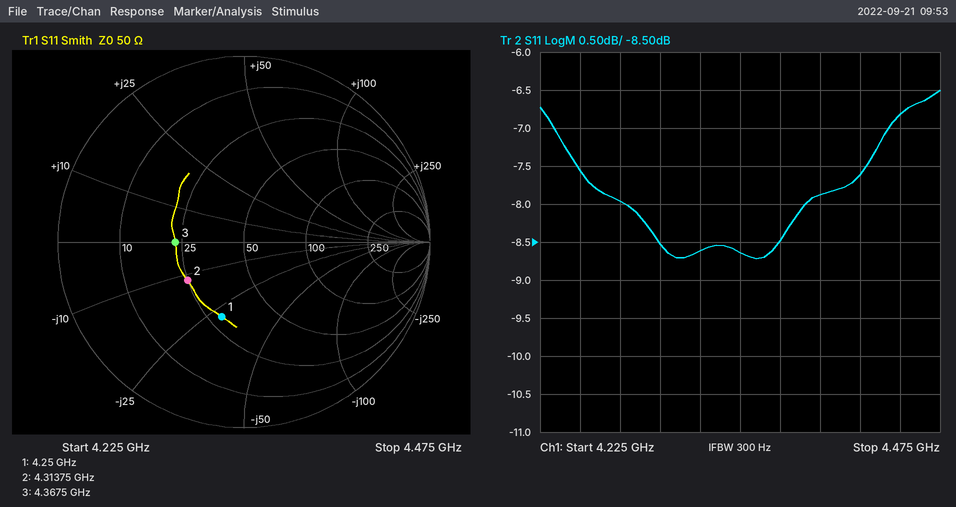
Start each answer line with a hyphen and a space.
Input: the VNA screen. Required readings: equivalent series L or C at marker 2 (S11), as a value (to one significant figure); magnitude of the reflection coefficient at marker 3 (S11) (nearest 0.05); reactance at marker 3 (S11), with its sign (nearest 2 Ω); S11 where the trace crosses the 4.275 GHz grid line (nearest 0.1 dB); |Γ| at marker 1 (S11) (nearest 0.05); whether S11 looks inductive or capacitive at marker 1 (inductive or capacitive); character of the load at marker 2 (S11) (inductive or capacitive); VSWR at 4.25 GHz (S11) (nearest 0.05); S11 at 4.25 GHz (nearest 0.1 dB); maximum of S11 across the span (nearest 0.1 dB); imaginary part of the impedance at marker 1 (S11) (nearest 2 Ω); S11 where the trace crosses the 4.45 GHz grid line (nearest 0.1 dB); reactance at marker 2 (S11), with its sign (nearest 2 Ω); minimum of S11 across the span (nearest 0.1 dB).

- 3 pF
- 0.35
- 0 Ω
- -8.0 dB
- 0.40
- capacitive
- capacitive
- 2.45
- -7.6 dB
- -6.5 dB
- -28 Ω
- -6.8 dB
- -12 Ω
- -8.7 dB
